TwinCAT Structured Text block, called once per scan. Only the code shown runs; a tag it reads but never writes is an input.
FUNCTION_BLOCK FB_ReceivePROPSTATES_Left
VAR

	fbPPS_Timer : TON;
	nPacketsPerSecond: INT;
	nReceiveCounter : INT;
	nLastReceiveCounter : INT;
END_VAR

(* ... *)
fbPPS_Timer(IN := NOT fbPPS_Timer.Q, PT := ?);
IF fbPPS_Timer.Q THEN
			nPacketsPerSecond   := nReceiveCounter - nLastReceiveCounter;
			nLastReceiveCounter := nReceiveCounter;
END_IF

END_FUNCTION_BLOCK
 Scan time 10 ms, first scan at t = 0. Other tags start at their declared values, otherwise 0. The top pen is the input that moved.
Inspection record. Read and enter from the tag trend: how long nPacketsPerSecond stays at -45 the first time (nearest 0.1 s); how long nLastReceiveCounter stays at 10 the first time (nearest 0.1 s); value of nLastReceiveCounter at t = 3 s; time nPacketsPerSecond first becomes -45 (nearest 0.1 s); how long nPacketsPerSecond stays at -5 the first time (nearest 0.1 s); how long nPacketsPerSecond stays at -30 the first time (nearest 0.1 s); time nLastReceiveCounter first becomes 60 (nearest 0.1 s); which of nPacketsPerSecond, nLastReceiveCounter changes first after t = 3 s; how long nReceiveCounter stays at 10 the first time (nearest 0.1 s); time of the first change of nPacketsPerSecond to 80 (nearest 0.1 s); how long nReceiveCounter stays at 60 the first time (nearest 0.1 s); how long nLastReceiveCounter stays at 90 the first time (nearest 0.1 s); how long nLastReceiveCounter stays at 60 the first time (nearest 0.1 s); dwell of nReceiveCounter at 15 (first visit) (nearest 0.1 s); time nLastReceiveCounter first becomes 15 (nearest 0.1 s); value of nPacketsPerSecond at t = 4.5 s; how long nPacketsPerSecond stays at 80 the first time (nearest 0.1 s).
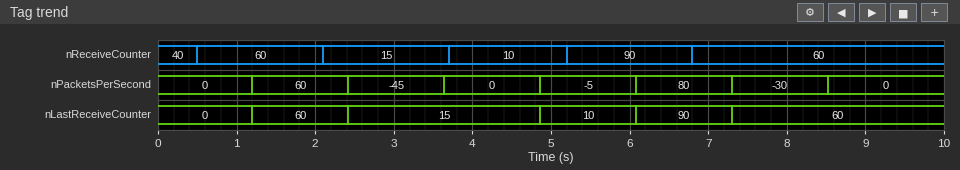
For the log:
1.2 s
1.2 s
15
2.4 s
1.2 s
1.2 s
1.2 s
nPacketsPerSecond
1.5 s
6.1 s
1.6 s
1.2 s
1.2 s
1.6 s
2.4 s
0
1.2 s
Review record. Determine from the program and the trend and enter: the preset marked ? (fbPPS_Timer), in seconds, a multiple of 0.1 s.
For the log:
1.2 s
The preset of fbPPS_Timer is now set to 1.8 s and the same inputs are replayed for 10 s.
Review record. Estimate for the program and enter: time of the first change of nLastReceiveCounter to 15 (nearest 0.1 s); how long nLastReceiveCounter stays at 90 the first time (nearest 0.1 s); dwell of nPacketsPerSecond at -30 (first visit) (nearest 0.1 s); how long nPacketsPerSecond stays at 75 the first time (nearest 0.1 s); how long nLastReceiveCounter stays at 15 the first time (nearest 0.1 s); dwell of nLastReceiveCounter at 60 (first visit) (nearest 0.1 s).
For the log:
3.6 s
1.8 s
1.8 s
1.8 s
1.8 s
1.8 s
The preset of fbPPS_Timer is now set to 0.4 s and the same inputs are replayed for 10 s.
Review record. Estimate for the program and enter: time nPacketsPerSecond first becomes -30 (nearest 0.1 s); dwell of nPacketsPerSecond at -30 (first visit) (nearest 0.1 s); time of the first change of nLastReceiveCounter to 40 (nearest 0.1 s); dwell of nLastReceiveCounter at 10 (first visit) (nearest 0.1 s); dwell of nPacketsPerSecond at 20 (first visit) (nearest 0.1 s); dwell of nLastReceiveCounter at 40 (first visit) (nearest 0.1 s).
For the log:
7.1 s
0.4 s
0.4 s
1.7 s
0.4 s
0.4 s
